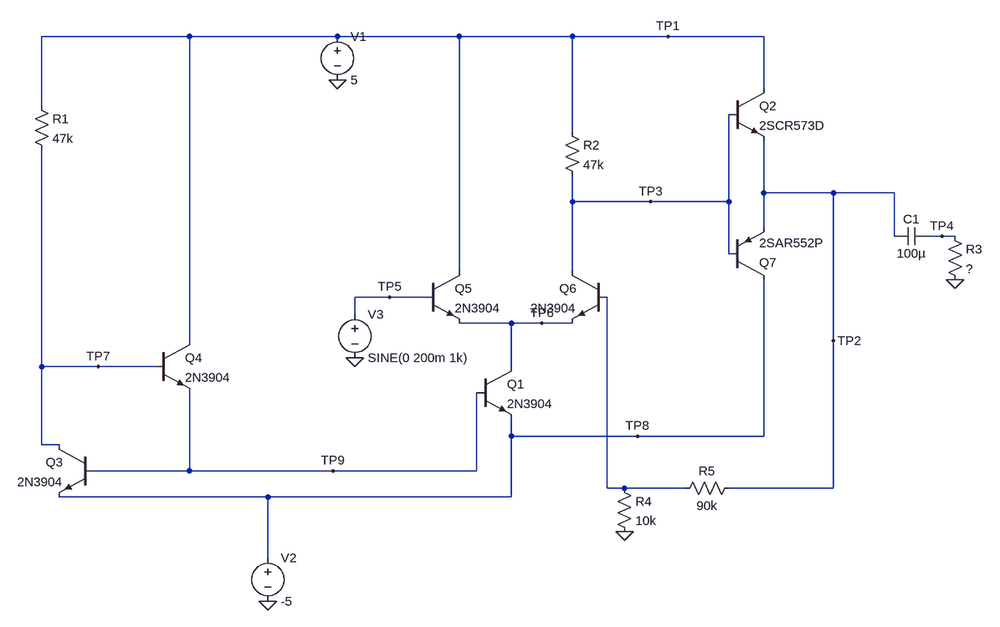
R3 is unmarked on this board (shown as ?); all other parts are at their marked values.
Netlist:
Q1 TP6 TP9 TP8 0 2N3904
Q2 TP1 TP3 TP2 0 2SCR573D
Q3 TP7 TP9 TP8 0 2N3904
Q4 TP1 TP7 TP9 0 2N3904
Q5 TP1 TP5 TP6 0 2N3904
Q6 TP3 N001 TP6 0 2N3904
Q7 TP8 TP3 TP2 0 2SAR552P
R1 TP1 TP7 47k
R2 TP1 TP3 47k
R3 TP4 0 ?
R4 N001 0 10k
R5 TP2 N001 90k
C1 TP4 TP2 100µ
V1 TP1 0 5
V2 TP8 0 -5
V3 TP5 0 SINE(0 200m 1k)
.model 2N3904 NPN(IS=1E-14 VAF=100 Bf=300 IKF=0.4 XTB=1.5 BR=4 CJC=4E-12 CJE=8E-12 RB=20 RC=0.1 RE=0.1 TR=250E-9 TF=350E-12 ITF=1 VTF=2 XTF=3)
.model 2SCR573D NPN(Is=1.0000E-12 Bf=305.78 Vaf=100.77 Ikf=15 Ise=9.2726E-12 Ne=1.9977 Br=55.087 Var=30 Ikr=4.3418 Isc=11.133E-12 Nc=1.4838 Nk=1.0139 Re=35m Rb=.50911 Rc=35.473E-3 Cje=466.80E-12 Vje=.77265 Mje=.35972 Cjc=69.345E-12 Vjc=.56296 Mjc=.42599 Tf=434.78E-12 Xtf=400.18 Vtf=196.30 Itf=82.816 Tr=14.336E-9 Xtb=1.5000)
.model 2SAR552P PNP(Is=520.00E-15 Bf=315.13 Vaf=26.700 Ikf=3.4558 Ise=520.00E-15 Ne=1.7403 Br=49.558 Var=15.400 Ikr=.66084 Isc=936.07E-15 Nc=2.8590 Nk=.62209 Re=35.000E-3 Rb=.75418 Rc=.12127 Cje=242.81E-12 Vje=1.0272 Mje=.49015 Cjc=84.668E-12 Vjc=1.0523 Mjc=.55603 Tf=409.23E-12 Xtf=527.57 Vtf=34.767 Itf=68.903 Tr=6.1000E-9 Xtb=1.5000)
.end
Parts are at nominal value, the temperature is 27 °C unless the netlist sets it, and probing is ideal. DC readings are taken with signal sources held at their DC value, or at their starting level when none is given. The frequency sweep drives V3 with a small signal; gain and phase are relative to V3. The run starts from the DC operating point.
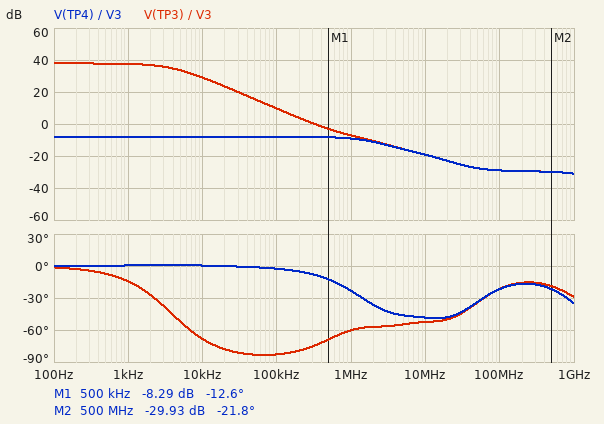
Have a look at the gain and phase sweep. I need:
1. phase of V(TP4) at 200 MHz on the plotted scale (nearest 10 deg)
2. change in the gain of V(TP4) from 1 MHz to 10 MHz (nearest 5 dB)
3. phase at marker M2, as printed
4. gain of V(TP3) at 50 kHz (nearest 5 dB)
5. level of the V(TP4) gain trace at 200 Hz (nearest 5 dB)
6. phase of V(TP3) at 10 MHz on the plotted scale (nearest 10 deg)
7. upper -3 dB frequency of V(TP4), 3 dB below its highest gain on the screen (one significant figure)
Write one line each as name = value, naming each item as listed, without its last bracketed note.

phase of V(TP4) at 200 MHz on the plotted scale = -20 deg
change in the gain of V(TP4) from 1 MHz to 10 MHz = -10 dB
phase at marker M2, as printed = -21.8 deg
gain of V(TP3) at 50 kHz = 15 dB
level of the V(TP4) gain trace at 200 Hz = -10 dB
phase of V(TP3) at 10 MHz on the plotted scale = -50 deg
upper -3 dB frequency of V(TP4), 3 dB below its highest gain on the screen = 2 MHz
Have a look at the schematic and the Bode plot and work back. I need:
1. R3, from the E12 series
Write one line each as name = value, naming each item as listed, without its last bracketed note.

R3, from the E12 series = 270 Ω
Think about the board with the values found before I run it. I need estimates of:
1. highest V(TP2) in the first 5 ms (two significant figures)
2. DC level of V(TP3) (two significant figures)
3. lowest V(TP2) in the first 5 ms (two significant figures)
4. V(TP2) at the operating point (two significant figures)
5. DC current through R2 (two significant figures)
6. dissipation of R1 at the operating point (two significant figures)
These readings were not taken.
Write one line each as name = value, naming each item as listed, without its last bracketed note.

highest V(TP2) in the first 5 ms = 1.7 V
DC level of V(TP3) = 380 mV
lowest V(TP2) in the first 5 ms = -200 mV
V(TP2) at the operating point = 45 mV
DC current through R2 = 98 µA
dissipation of R1 at the operating point = 1.7 mW
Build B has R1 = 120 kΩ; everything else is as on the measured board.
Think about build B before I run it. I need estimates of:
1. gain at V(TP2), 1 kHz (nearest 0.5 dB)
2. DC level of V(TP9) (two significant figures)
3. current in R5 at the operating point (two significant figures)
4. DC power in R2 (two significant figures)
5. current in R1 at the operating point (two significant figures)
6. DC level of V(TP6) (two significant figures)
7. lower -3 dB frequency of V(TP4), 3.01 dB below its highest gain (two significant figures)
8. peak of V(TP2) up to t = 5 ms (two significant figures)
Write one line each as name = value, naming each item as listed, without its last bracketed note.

gain at V(TP2), 1 kHz = -12.5 dB
DC level of V(TP9) = -4.4 V
current in R5 at the operating point = 10 µA
DC power in R2 = 270 µW
current in R1 at the operating point = 75 µA
DC level of V(TP6) = -490 mV
lower -3 dB frequency of V(TP4), 3.01 dB below its highest gain = 680 mHz
peak of V(TP2) up to t = 5 ms = 2.0 V
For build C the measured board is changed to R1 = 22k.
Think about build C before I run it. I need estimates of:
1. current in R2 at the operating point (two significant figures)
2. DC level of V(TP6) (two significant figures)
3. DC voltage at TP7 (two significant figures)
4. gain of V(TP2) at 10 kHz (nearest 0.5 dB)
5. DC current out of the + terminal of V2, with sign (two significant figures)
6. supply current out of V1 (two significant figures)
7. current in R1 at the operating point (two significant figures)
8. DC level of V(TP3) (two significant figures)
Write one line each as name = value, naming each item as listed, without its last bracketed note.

current in R2 at the operating point = 120 µA
DC level of V(TP6) = -620 mV
DC voltage at TP7 = -3.9 V
gain of V(TP2) at 10 kHz = -20.0 dB
DC current out of the + terminal of V2, with sign = -820 µA
supply current out of V1 = 820 µA
current in R1 at the operating point = 400 µA
DC level of V(TP3) = -520 mV
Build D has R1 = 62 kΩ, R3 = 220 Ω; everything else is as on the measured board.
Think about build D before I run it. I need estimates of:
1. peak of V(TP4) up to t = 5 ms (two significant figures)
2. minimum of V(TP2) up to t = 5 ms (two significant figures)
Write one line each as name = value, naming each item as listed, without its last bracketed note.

peak of V(TP4) up to t = 5 ms = 1.5 V
minimum of V(TP2) up to t = 5 ms = -140 mV
